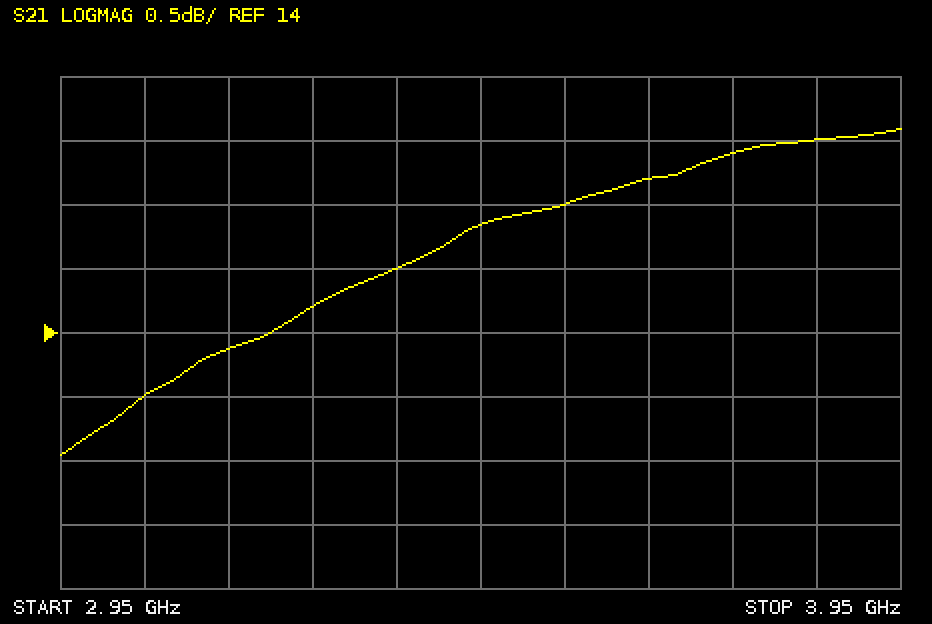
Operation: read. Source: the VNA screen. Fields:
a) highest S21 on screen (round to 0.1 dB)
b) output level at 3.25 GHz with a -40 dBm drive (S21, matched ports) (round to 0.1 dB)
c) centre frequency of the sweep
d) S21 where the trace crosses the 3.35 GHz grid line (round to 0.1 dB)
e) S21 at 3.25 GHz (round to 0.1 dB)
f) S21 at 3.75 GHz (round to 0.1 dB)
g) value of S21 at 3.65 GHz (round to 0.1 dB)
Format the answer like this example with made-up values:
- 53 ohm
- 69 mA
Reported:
- 15.6 dB
- -25.8 dBm
- 3.45 GHz
- 14.5 dB
- 14.2 dB
- 15.4 dB
- 15.2 dB
